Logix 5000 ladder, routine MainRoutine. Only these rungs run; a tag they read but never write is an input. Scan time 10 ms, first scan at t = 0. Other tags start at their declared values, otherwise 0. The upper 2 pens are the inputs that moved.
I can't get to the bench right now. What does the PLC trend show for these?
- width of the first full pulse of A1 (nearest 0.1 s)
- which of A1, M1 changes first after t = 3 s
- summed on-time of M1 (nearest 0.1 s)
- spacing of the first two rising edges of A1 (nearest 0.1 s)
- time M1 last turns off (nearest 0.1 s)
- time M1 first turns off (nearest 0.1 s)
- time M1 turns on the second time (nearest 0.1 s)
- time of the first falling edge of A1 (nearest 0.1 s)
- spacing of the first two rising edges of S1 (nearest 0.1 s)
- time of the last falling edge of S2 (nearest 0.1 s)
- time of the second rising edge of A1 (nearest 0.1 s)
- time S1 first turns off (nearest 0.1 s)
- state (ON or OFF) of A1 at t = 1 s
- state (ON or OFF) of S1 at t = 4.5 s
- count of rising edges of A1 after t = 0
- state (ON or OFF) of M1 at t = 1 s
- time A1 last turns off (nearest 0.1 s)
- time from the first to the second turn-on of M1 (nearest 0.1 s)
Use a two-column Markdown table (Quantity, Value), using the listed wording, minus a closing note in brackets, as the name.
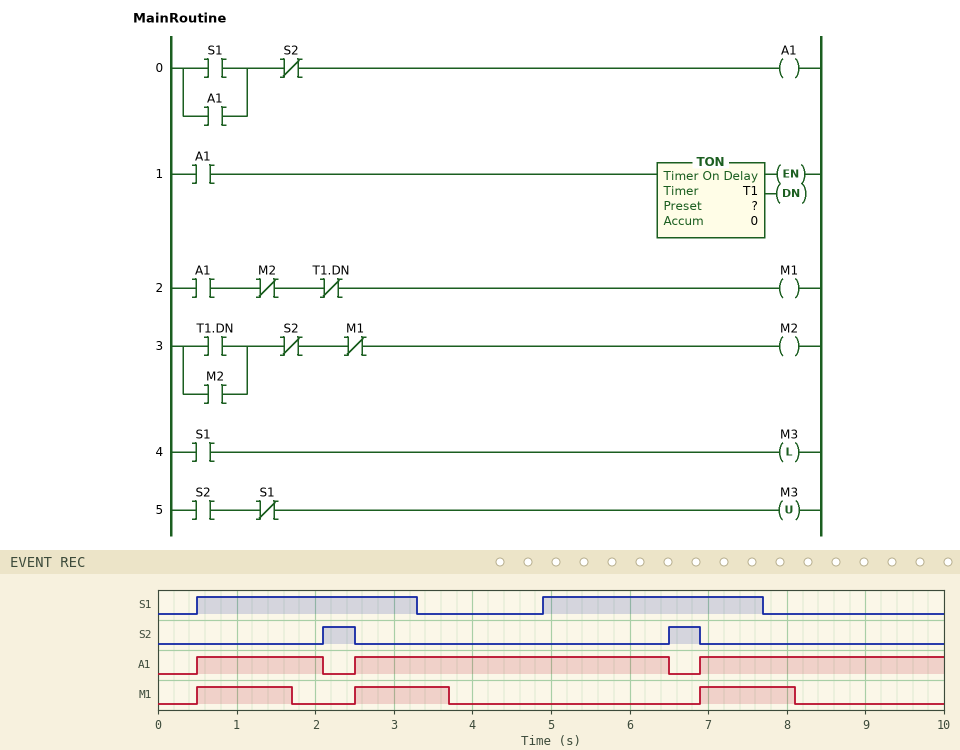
| Quantity | Value |
|---|---|
| width of the first full pulse of A1 | 1.6 s |
| which of A1, M1 changes first after t = 3 s | M1 |
| summed on-time of M1 | 3.6 s |
| spacing of the first two rising edges of A1 | 2.0 s |
| time M1 last turns off | 8.1 s |
| time M1 first turns off | 1.7 s |
| time M1 turns on the second time | 2.5 s |
| time of the first falling edge of A1 | 2.1 s |
| spacing of the first two rising edges of S1 | 4.4 s |
| time of the last falling edge of S2 | 6.9 s |
| time of the second rising edge of A1 | 2.5 s |
| time S1 first turns off | 3.3 s |
| state (ON or OFF) of A1 at t = 1 s | ON |
| state (ON or OFF) of S1 at t = 4.5 s | OFF |
| count of rising edges of A1 after t = 0 | 3 |
| state (ON or OFF) of M1 at t = 1 s | ON |
| time A1 last turns off | 6.5 s |
| time from the first to the second turn-on of M1 | 2.0 s |
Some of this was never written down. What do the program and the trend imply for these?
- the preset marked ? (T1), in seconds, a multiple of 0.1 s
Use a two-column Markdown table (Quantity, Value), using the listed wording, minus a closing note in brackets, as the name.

| Quantity | Value |
|---|---|
| the preset marked ? (T1), in seconds, a multiple of 0.1 s | 1.2 s |
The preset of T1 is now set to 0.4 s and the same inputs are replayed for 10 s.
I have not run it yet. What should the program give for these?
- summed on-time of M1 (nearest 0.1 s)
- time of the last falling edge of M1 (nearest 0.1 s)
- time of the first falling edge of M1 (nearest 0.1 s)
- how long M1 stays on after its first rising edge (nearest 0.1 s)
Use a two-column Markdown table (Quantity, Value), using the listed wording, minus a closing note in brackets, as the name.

| Quantity | Value |
|---|---|
| summed on-time of M1 | 1.2 s |
| time of the last falling edge of M1 | 7.3 s |
| time of the first falling edge of M1 | 0.9 s |
| how long M1 stays on after its first rising edge | 0.4 s |
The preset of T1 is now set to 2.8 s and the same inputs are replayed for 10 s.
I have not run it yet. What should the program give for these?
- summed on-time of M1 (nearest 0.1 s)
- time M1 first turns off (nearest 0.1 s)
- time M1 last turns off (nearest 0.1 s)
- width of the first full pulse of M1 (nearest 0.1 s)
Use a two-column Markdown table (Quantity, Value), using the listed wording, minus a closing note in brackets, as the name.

| Quantity | Value |
|---|---|
| summed on-time of M1 | 7.2 s |
| time M1 first turns off | 2.1 s |
| time M1 last turns off | 9.7 s |
| width of the first full pulse of M1 | 1.6 s |
